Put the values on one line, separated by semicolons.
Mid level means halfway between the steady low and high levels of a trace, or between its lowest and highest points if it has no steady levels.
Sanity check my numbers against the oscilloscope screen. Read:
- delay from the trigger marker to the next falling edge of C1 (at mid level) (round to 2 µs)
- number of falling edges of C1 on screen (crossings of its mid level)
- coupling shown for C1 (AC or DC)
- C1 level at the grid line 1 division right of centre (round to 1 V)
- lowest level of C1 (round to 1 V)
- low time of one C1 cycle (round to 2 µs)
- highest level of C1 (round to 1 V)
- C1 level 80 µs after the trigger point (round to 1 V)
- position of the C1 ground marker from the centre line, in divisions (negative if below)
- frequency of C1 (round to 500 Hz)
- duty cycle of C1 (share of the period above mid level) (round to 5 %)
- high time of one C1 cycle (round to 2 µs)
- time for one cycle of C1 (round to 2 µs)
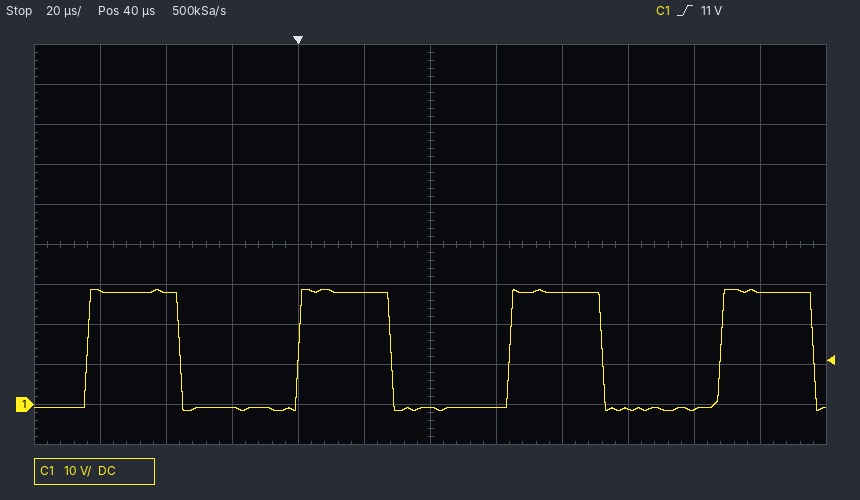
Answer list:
28 µs; 4; DC; -1 V; -2 V; 36 µs; 29 V; 28 V; -4.0 div; 15.5 kHz; 45 %; 28 µs; 64 µs
